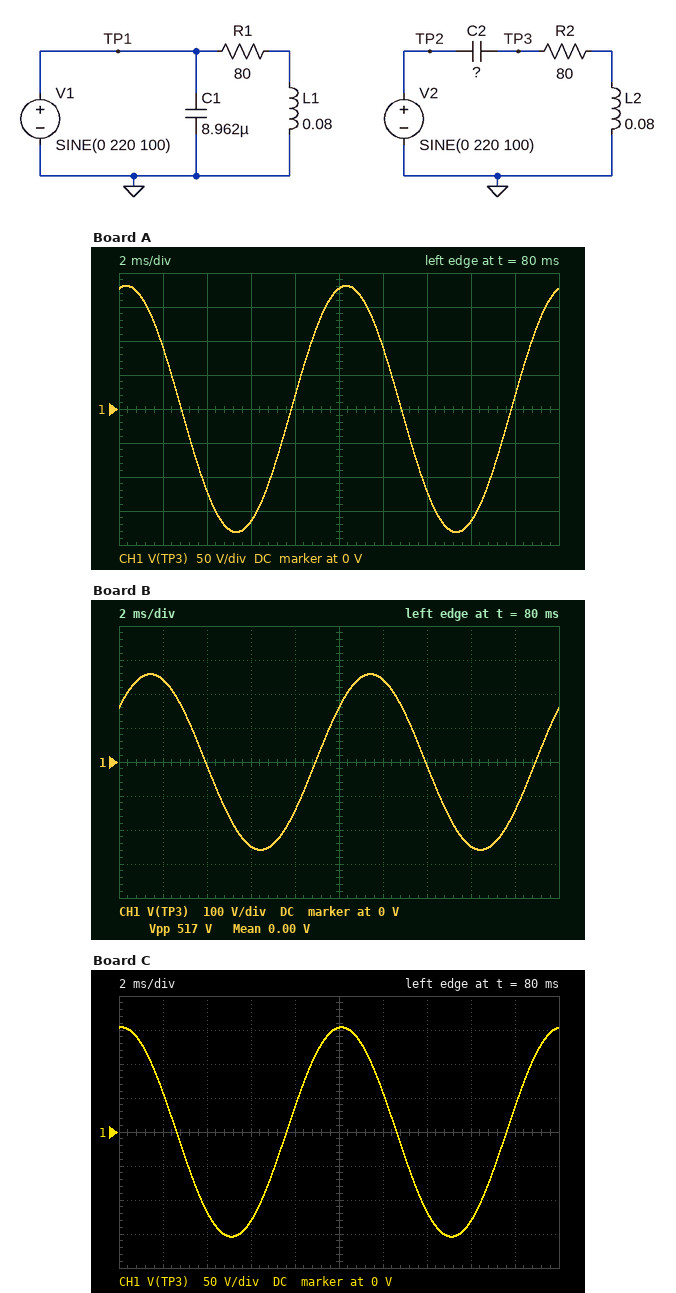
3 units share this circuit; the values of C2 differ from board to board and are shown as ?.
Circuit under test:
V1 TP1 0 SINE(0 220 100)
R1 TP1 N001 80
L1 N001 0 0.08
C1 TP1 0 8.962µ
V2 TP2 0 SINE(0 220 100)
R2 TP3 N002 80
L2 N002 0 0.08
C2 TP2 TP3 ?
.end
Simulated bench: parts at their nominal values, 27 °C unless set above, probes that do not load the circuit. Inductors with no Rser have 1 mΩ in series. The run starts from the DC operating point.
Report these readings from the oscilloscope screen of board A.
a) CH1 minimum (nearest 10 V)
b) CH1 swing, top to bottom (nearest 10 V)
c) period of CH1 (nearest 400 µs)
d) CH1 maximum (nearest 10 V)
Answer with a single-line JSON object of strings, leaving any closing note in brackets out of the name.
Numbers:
{"CH1 minimum": "-180 V", "CH1 swing, top to bottom": "360 V", "period of CH1": "10.0 ms", "CH1 maximum": "180 V"}
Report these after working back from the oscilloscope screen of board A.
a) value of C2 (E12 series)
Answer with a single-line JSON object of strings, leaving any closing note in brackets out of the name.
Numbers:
{"value of C2": "12 µF"}
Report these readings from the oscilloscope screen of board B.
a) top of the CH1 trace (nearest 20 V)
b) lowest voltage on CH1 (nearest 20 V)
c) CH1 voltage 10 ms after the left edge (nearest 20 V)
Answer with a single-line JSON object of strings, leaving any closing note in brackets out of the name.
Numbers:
{"top of the CH1 trace": "260 V", "lowest voltage on CH1": "-260 V", "CH1 voltage 10 ms after the left edge": "160 V"}
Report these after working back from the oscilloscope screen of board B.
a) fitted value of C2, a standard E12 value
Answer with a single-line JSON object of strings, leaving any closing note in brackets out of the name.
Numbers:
{"fitted value of C2, a standard E12 value": "27 µF"}
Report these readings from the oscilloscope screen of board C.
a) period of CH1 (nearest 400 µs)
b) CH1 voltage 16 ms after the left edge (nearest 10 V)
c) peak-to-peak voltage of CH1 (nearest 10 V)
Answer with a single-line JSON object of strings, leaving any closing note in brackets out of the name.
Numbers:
{"period of CH1": "10.0 ms", "CH1 voltage 16 ms after the left edge": "-130 V", "peak-to-peak voltage of CH1": "310 V"}
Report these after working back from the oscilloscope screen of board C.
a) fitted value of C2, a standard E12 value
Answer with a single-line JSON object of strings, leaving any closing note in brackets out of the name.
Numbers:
{"fitted value of C2, a standard E12 value": "10 µF"}
